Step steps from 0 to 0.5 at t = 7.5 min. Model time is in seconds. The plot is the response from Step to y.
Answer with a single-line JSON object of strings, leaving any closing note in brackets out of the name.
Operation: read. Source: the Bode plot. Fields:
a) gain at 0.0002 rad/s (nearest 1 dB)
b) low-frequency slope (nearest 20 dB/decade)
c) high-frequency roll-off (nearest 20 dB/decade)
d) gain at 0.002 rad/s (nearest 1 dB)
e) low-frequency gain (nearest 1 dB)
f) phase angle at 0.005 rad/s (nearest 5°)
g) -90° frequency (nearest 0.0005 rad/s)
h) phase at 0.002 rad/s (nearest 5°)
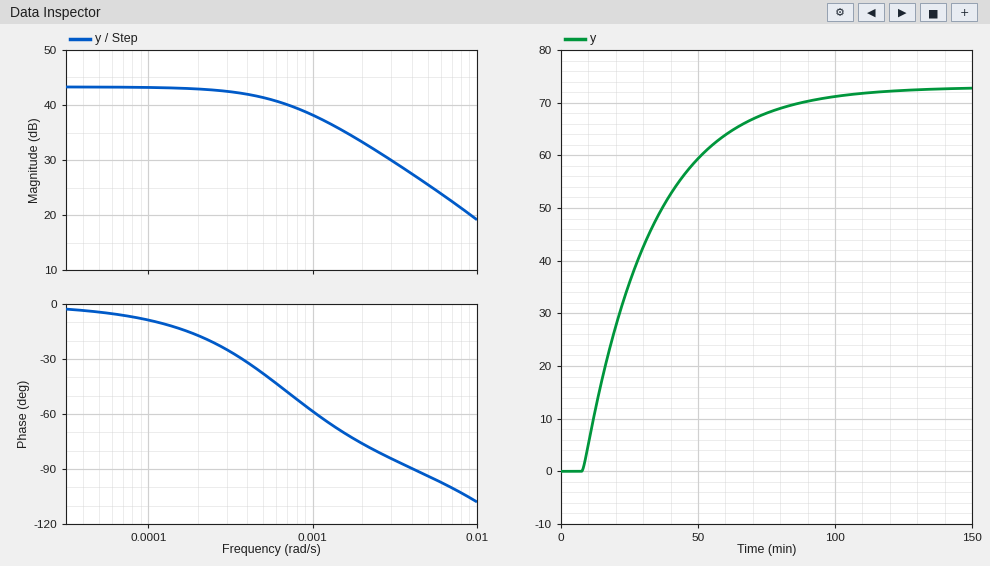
{"gain at 0.0002 rad/s": "43 dB", "low-frequency slope": "0 dB/decade", "high-frequency roll-off": "-20 dB/decade", "gain at 0.002 rad/s": "33 dB", "low-frequency gain": "43 dB", "phase angle at 0.005 rad/s": "-95°", "-90° frequency": "0.0040 rad/s", "phase at 0.002 rad/s": "-75°"}
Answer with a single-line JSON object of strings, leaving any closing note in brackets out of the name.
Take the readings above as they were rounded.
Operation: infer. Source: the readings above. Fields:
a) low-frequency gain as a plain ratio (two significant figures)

{"low-frequency gain as a plain ratio": "140"}
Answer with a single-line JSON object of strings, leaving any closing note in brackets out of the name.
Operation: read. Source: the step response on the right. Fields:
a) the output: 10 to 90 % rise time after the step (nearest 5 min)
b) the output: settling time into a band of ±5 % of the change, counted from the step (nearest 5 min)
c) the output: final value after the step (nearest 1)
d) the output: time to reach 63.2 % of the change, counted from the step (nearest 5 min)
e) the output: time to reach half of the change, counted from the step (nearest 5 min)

{"the output: 10 to 90 % rise time after the step": "55 min", "the output: settling time into a band of ±5 % of the change, counted from the step": "75 min", "the output: final value after the step": "73", "the output: time to reach 63.2 % of the change, counted from the step": "25 min", "the output: time to reach half of the change, counted from the step": "20 min"}
